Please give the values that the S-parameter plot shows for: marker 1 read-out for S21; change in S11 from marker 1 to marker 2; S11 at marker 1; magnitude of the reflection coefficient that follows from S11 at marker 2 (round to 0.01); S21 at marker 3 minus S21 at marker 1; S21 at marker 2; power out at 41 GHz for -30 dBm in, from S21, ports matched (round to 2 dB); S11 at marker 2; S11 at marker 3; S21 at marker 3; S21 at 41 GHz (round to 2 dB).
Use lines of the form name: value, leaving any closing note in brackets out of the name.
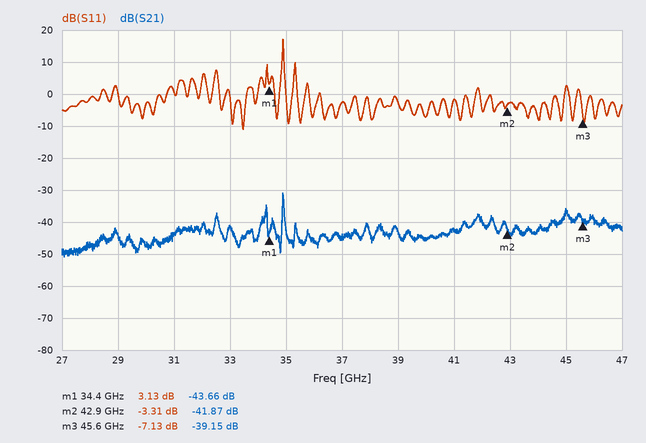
marker 1 read-out for S21: -43.66 dB
change in S11 from marker 1 to marker 2: -6.44 dB
S11 at marker 1: 3.13 dB
magnitude of the reflection coefficient that follows from S11 at marker 2: 0.68
S21 at marker 3 minus S21 at marker 1: 4.51 dB
S21 at marker 2: -41.87 dB
power out at 41 GHz for -30 dBm in, from S21, ports matched: -72 dBm
S11 at marker 2: -3.31 dB
S11 at marker 3: -7.13 dB
S21 at marker 3: -39.15 dB
S21 at 41 GHz: -42 dB
